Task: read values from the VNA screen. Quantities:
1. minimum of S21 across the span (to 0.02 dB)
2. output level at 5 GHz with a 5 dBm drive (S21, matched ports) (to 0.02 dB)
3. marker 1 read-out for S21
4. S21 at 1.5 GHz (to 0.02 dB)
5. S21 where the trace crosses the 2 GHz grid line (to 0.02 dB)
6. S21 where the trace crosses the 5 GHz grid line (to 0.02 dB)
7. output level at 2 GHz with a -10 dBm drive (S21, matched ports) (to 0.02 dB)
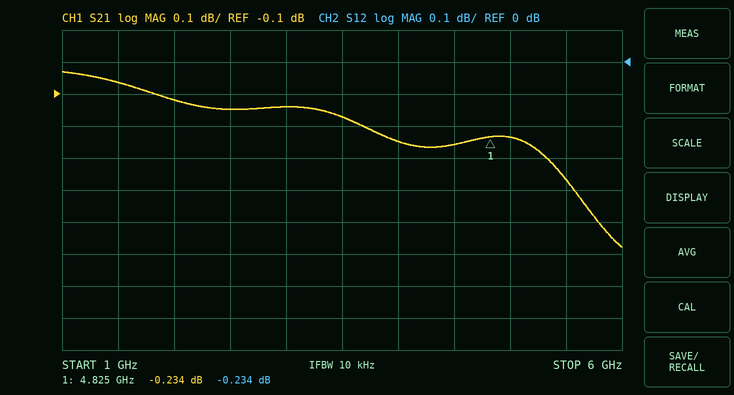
-0.58 dB
4.76 dBm
-0.234 dB
-0.06 dB
-0.12 dB
-0.24 dB
-10.12 dBm
